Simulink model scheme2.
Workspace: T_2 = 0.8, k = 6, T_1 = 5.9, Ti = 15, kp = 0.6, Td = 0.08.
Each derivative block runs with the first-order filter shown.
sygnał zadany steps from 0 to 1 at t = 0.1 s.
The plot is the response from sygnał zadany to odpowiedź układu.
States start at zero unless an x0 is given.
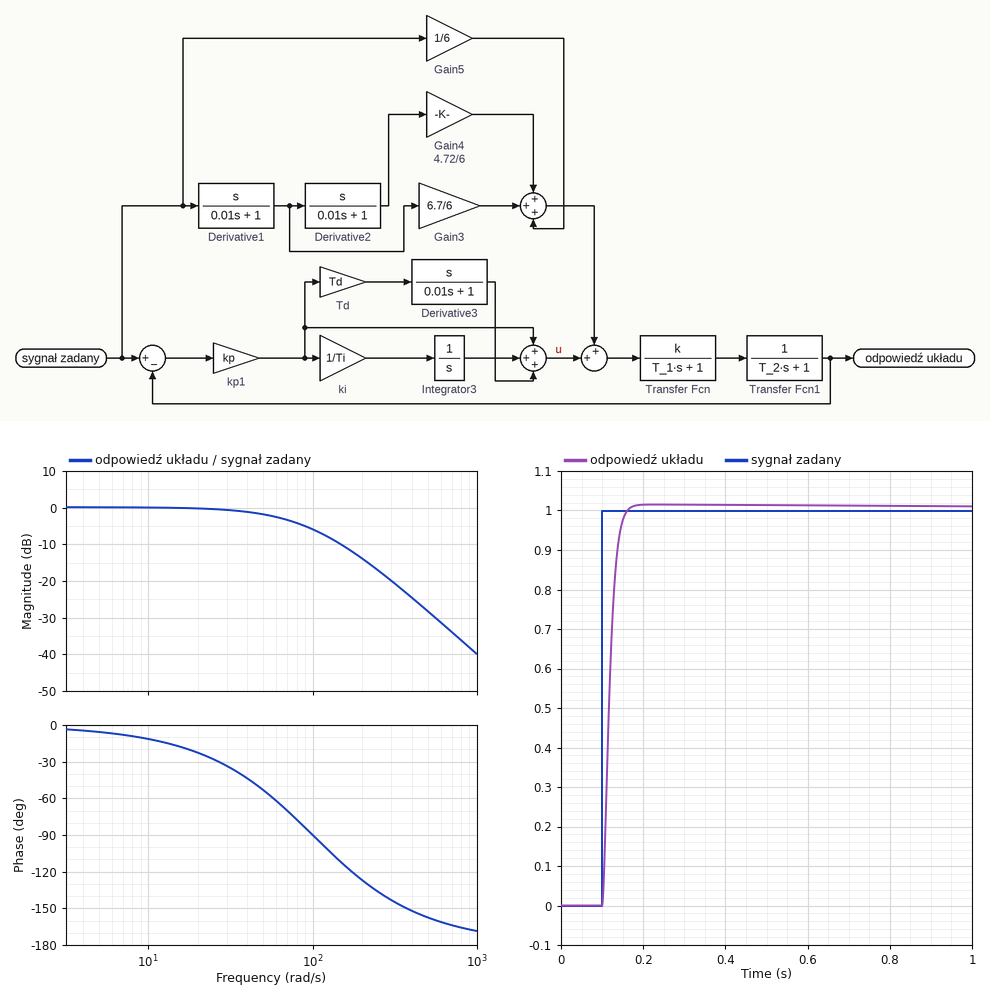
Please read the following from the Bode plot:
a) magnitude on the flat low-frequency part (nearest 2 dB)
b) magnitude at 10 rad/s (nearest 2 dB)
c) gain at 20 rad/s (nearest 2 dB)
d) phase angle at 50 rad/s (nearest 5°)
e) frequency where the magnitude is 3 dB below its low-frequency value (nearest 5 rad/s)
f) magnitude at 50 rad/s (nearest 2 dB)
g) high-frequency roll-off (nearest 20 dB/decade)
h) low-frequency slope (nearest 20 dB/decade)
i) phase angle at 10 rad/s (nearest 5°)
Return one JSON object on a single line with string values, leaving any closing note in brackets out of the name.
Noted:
{"magnitude on the flat low-frequency part": "0 dB", "magnitude at 10 rad/s": "0 dB", "gain at 20 rad/s": "0 dB", "phase angle at 50 rad/s": "-55°", "frequency where the magnitude is 3 dB below its low-frequency value": "65 rad/s", "magnitude at 50 rad/s": "-2 dB", "high-frequency roll-off": "-40 dB/decade", "low-frequency slope": "0 dB/decade", "phase angle at 10 rad/s": "-10°"}
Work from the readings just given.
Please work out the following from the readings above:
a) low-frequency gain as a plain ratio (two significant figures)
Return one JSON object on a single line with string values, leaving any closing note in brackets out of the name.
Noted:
{"low-frequency gain as a plain ratio": "1.0"}
